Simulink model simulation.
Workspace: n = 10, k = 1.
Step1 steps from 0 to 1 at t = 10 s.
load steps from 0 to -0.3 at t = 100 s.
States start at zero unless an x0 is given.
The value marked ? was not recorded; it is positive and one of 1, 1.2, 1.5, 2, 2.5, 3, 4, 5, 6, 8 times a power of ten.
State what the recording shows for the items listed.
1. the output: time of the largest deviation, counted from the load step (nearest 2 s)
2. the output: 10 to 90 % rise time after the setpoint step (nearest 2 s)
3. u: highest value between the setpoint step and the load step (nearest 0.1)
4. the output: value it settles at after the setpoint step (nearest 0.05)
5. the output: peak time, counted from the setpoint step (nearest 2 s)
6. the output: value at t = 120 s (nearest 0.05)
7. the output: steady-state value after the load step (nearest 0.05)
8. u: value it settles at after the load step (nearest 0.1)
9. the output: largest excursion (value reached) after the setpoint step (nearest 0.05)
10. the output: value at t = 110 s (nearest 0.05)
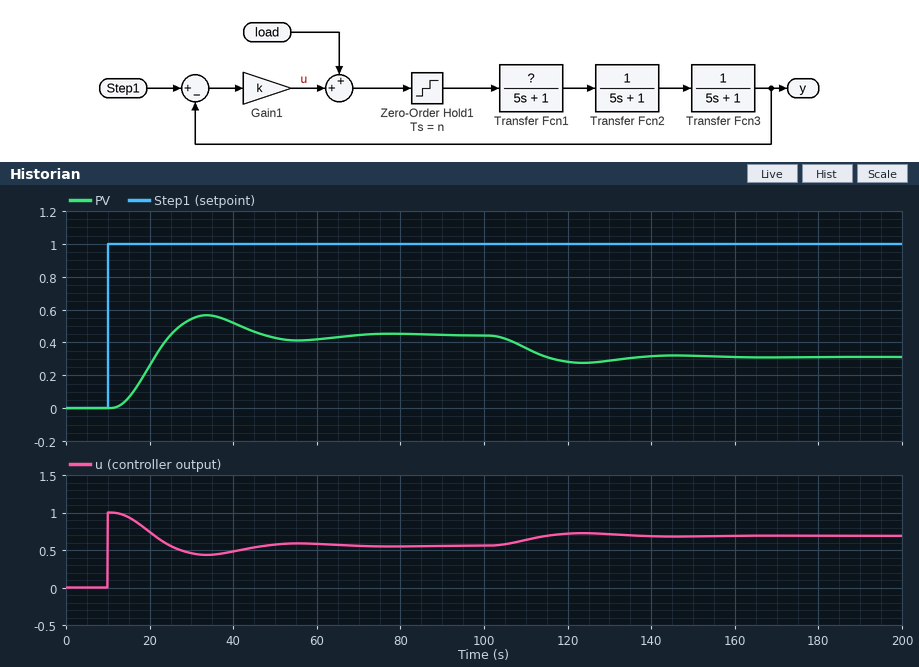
24 s
10 s
1.0
0.45
24 s
0.30
0.30
0.7
0.55
0.35
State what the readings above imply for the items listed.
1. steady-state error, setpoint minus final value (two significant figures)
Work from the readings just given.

0.55
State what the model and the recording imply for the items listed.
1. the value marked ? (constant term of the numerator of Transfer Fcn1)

0.8
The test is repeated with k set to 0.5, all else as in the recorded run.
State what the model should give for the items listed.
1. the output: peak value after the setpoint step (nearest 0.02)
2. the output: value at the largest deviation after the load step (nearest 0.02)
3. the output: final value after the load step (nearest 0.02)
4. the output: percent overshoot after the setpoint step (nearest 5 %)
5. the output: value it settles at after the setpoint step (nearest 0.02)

0.32
0.10
0.12
10 %
0.28
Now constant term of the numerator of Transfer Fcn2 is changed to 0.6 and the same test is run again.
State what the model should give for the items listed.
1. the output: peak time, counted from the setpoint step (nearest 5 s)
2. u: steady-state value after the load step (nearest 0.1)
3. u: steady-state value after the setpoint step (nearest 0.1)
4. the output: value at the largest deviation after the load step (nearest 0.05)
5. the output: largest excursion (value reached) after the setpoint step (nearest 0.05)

25 s
0.8
0.7
0.20
0.35
